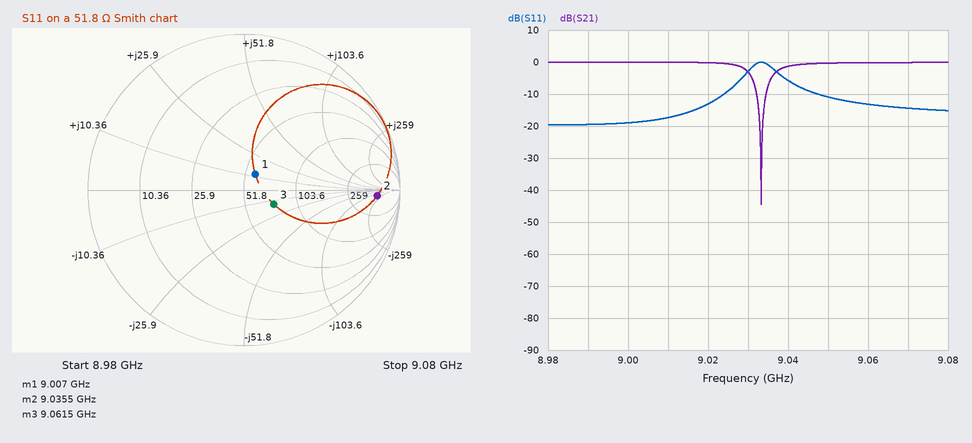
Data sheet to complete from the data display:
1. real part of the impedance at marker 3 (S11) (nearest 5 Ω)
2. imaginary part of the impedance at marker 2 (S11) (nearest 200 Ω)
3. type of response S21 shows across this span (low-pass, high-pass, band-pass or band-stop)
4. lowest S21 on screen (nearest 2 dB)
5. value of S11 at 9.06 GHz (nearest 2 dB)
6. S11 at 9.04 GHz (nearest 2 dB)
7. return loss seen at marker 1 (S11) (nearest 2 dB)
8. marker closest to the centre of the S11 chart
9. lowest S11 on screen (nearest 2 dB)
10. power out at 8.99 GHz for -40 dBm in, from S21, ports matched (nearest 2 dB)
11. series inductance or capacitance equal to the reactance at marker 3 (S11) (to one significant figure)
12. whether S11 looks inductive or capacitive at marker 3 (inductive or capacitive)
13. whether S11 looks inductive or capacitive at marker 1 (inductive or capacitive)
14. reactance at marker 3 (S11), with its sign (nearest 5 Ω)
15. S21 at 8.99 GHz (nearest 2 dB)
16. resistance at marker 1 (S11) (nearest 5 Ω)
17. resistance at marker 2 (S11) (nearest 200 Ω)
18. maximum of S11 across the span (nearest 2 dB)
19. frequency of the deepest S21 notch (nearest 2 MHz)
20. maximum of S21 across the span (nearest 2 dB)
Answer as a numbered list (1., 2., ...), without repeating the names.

1. 75 Ω
2. -200 Ω
3. band-stop
4. -44 dB
5. -14 dB
6. -6 dB
7. 18 dB
8. marker 1
9. -20 dB
10. -40 dBm
11. 1 pF
12. capacitive
13. inductive
14. -15 Ω
15. 0 dB
16. 60 Ω
17. 600 Ω
18. 0 dB
19. 9.034 GHz
20. 0 dB
